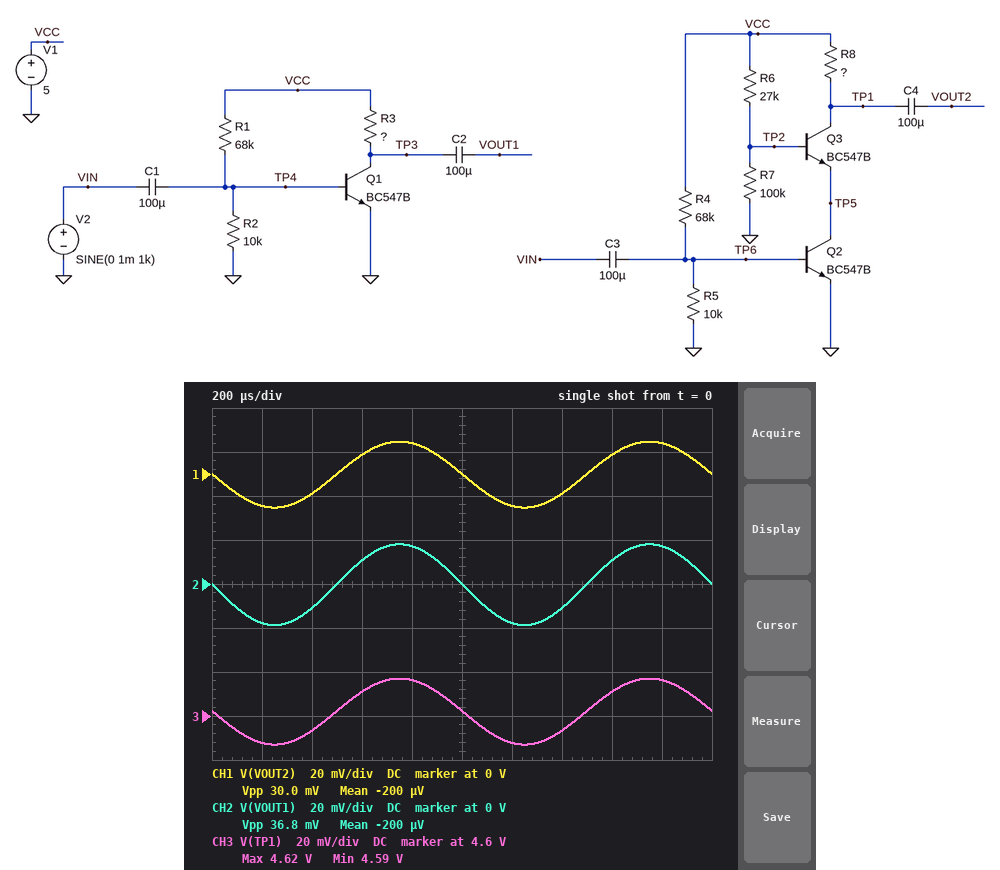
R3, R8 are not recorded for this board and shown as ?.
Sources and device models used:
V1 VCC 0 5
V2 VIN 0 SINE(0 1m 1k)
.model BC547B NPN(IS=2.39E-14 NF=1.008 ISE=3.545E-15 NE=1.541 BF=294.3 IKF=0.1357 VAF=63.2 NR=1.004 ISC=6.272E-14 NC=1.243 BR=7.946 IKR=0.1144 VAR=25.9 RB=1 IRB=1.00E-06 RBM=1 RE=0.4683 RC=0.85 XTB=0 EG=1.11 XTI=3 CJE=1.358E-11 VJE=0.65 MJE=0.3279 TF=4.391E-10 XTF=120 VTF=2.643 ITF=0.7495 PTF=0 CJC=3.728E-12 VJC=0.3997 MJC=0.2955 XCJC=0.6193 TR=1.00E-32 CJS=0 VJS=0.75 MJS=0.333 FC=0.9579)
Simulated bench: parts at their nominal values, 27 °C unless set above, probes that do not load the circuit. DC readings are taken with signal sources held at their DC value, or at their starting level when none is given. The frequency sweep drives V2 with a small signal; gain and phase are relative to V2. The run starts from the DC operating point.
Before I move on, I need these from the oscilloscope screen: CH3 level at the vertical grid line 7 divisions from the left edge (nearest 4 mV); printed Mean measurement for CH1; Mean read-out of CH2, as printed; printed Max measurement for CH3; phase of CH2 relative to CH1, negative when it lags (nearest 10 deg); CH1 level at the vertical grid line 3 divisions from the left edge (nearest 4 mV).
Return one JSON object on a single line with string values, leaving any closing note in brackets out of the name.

{"CH3 level at the vertical grid line 7 divisions from the left edge": "4.592 V", "printed Mean measurement for CH1": "-200 µV", "Mean read-out of CH2, as printed": "-200 µV", "printed Max measurement for CH3": "4.62 V", "phase of CH2 relative to CH1, negative when it lags": "0 deg", "CH1 level at the vertical grid line 3 divisions from the left edge": "8 mV"}
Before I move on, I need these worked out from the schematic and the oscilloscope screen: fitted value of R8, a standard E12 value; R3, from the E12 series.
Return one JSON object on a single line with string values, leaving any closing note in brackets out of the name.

{"fitted value of R8, a standard E12 value": "680 Ω", "R3, from the E12 series": "820 Ω"}
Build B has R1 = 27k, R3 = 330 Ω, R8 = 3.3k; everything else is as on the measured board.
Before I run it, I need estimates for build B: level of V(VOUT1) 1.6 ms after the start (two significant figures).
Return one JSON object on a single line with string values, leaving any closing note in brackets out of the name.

{"level of V(VOUT1) 1.6 ms after the start": "49 mV"}
